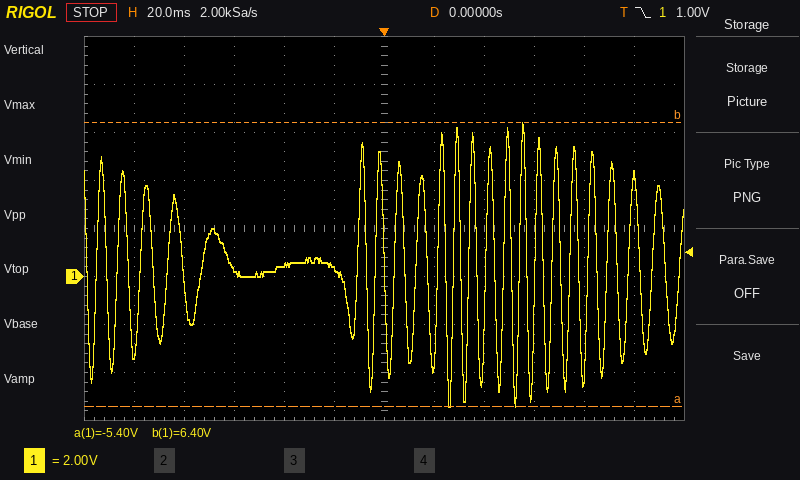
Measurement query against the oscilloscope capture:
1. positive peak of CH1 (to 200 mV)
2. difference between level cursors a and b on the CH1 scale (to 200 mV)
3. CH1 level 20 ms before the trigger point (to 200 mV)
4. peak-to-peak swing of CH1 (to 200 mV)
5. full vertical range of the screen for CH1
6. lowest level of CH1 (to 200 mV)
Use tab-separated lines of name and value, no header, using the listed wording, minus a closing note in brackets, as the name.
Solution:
positive peak of CH1	6.4 V
difference between level cursors a and b on the CH1 scale	11.8 V
CH1 level 20 ms before the trigger point	400 mV
peak-to-peak swing of CH1	11.8 V
full vertical range of the screen for CH1	16 V
lowest level of CH1	-5.4 V
